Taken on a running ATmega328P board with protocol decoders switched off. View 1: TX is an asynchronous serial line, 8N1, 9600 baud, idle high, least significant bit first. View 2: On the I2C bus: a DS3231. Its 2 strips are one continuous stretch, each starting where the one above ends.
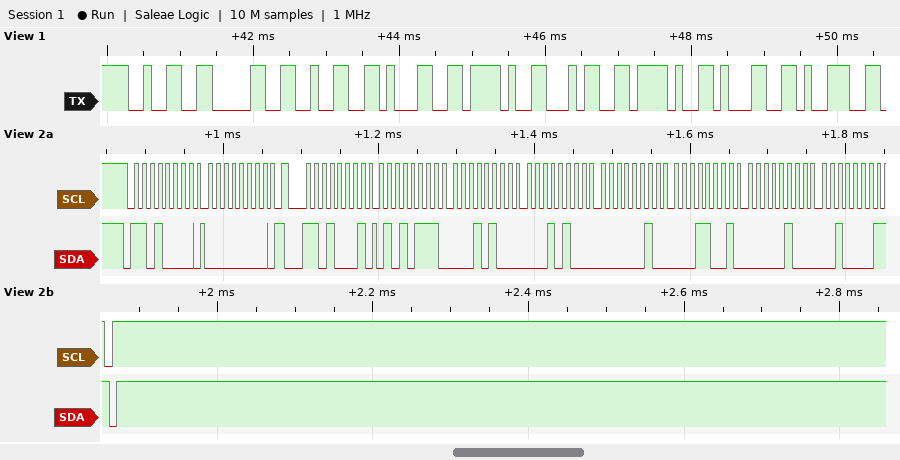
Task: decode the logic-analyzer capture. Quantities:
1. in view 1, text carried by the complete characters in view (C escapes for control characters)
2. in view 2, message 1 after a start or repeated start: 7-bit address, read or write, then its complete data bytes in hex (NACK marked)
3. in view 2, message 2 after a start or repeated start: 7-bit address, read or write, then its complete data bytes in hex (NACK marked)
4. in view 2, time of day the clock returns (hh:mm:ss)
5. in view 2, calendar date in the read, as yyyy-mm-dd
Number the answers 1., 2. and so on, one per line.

1. "2021/4/19"
2. 0x68 write: 00
3. 0x68 read: 57 14 14 02 19 04 21 NACK
4. 14:14:57
5. 2021-04-19
